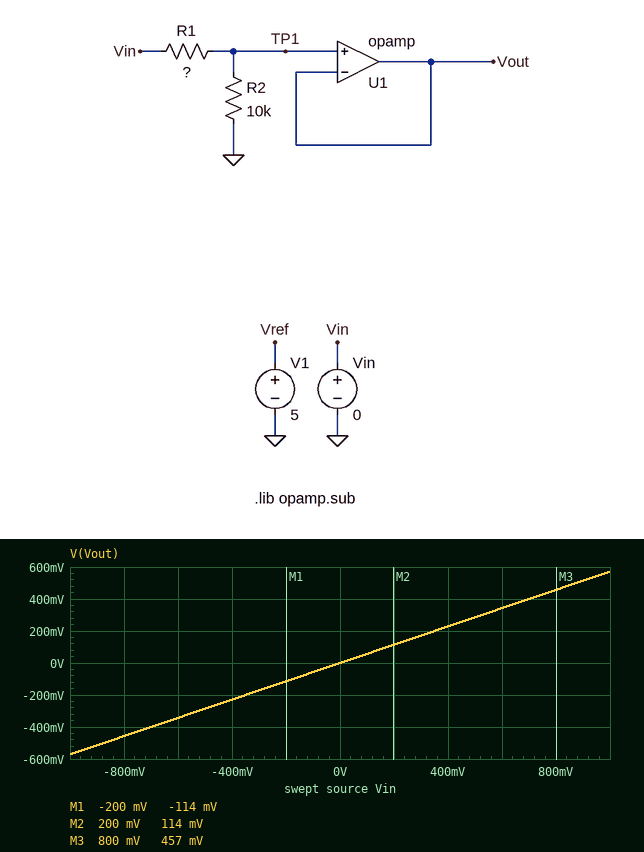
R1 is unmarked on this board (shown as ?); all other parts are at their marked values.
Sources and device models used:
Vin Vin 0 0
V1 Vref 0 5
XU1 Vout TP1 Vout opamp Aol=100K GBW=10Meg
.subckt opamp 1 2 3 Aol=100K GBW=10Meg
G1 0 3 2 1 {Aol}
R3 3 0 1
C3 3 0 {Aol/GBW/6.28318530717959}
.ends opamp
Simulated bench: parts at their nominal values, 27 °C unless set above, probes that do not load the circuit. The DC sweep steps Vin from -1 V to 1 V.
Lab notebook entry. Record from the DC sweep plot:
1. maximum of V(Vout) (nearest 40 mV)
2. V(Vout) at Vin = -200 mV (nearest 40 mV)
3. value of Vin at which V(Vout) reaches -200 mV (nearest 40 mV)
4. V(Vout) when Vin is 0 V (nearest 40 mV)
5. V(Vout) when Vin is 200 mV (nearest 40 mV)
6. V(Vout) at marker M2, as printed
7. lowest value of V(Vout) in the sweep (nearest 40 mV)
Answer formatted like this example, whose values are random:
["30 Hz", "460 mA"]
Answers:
["560 mV", "-120 mV", "-360 mV", "0 V", "120 mV", "114 mV", "-560 mV"]
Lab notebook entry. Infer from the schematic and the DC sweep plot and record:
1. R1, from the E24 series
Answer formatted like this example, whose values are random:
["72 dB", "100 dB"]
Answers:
["7.5 kΩ"]
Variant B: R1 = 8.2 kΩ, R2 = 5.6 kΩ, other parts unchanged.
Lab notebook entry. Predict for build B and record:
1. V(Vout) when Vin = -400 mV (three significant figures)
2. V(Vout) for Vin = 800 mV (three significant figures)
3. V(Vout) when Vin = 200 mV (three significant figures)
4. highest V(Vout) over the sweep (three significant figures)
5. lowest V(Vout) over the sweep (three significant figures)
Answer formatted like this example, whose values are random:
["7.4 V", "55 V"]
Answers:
["-162 mV", "325 mV", "81.2 mV", "406 mV", "-406 mV"]
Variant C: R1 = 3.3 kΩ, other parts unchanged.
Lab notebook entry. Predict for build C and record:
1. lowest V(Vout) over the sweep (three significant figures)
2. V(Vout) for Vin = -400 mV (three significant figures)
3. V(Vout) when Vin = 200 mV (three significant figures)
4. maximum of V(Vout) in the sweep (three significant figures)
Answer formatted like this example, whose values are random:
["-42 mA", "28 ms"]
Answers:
["-752 mV", "-301 mV", "150 mV", "752 mV"]
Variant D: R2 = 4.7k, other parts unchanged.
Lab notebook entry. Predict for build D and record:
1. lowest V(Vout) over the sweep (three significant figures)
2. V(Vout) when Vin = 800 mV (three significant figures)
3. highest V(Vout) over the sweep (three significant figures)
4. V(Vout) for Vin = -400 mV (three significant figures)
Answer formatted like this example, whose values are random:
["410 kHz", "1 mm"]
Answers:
["-385 mV", "308 mV", "385 mV", "-154 mV"]
